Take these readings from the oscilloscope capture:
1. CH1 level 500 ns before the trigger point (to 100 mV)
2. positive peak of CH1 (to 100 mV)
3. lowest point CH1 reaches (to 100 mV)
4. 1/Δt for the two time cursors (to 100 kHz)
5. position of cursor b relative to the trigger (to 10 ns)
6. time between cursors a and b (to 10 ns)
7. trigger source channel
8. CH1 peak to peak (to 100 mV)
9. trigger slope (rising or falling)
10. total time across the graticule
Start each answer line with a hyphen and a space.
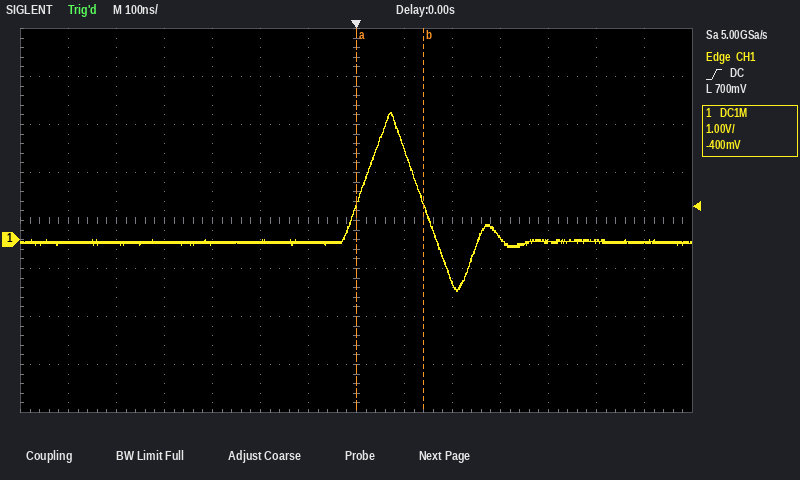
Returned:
- -100 mV
- 2.6 V
- -1.1 V
- 7.1 MHz
- +140 ns
- 140 ns
- CH1
- 3.7 V
- rising
- 1.4 µs
